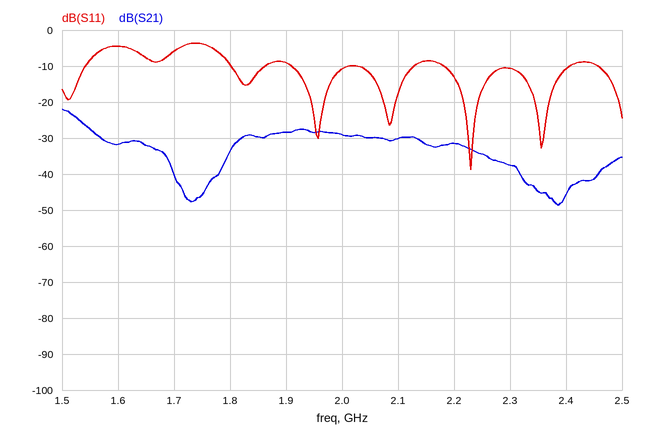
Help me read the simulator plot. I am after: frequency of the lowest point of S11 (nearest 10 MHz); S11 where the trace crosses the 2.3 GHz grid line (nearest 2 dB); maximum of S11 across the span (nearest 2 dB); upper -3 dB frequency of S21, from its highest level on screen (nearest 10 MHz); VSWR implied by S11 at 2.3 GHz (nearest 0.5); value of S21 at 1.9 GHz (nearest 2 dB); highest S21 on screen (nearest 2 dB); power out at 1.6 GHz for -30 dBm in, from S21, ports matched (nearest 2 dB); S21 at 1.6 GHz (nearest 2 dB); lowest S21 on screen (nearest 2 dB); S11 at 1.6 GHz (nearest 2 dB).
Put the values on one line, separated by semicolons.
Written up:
2.23 GHz; -10 dB; -4 dB; 1.53 GHz; 2.0; -28 dB; -22 dB; -62 dBm; -32 dB; -48 dB; -4 dB
